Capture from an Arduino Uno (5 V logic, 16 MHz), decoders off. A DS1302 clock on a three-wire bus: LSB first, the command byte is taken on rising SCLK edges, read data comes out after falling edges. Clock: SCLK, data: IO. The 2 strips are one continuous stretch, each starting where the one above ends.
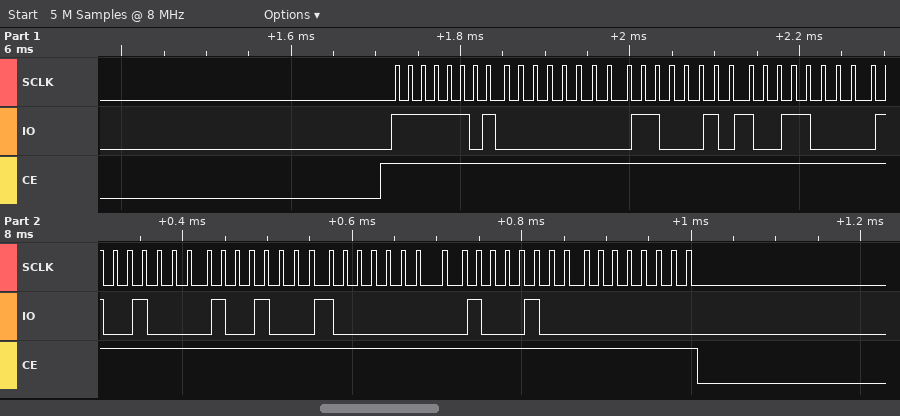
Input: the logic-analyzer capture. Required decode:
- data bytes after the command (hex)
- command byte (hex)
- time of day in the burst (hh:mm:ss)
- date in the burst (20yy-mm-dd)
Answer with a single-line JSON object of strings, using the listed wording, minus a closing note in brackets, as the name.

{"data bytes after the command": "00 46 19 12 12 01 22 00", "command byte": "0xBF", "time of day in the burst": "19:46:00", "date in the burst": "2022-12-12"}
